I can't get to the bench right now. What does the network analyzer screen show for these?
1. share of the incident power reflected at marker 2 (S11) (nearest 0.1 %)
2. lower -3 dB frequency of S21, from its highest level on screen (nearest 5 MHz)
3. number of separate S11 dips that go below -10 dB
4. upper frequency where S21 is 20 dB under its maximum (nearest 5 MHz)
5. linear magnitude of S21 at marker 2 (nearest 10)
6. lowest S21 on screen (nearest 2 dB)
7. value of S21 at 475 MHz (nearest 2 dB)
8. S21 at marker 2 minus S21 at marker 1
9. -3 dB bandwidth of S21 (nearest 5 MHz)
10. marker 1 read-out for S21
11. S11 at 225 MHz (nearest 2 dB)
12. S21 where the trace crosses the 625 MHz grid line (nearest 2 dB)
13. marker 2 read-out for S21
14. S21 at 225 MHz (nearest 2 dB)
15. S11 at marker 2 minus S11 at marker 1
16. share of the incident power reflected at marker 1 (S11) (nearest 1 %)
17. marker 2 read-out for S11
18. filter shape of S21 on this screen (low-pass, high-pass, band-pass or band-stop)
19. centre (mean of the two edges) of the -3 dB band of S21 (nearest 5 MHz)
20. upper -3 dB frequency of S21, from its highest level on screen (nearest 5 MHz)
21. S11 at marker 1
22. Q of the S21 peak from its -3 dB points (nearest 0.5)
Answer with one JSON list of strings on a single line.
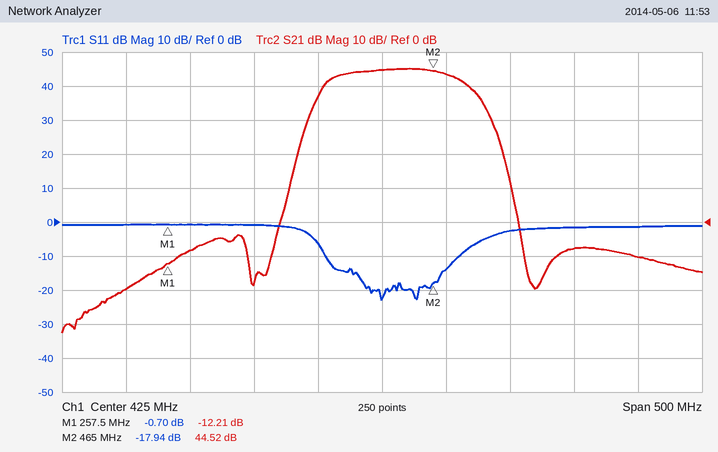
["1.6 %", "385 MHz", "2", "515 MHz", "170", "-32 dB", "44 dB", "56.73 dB", "100 MHz", "-12.21 dB", "0 dB", "-10 dB", "44.52 dB", "-20 dB", "-17.24 dB", "85 %", "-17.94 dB", "band-pass", "435 MHz", "485 MHz", "-0.70 dB", "4.5"]
